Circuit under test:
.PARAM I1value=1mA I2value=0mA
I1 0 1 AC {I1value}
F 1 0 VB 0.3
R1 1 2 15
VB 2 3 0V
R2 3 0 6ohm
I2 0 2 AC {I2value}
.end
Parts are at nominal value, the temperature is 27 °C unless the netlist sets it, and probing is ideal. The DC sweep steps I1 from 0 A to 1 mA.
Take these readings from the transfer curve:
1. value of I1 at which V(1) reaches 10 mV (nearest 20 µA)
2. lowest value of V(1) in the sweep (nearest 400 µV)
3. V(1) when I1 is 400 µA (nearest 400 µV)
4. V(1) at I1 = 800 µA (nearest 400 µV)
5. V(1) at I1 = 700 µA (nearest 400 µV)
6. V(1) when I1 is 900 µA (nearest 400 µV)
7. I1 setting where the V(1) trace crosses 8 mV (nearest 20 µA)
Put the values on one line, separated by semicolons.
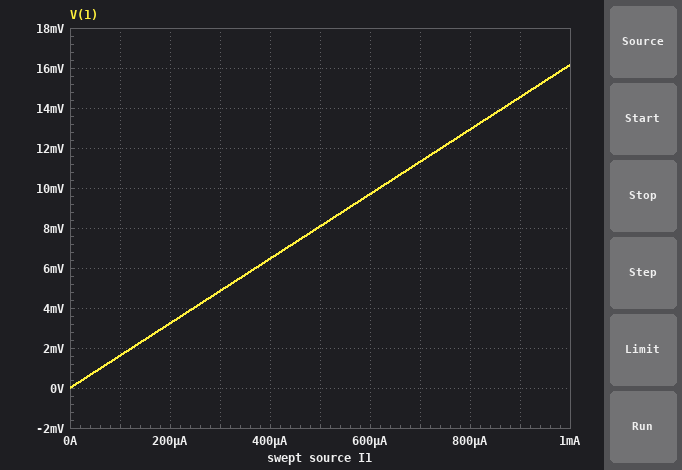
620 µA; 0 V; 6.4 mV; 12.8 mV; 11.2 mV; 14.4 mV; 500 µA
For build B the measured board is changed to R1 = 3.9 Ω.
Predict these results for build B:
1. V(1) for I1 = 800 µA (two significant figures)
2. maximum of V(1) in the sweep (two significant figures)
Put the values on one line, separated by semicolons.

6.1 mV; 7.6 mV
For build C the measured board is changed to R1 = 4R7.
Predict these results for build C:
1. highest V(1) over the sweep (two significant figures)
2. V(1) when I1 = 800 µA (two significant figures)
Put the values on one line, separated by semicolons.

8.2 mV; 6.6 mV
